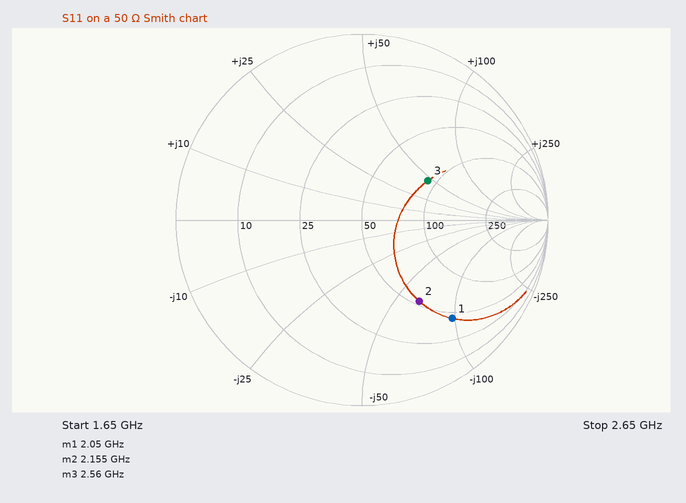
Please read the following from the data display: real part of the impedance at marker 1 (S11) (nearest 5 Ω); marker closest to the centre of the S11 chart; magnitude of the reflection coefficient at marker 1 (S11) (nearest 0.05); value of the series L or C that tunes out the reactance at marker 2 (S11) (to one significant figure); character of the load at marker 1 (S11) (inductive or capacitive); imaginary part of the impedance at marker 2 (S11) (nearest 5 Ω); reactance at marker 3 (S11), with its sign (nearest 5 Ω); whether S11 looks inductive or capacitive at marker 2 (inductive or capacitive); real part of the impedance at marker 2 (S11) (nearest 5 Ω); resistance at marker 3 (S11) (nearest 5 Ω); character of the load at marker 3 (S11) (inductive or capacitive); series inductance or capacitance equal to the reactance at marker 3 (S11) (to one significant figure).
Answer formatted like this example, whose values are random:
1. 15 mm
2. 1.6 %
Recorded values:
1. 45 Ω
2. marker 3
3. 0.70
4. 5 nH
5. capacitive
6. -65 Ω
7. +45 Ω
8. capacitive
9. 55 Ω
10. 90 Ω
11. inductive
12. 3 nH
